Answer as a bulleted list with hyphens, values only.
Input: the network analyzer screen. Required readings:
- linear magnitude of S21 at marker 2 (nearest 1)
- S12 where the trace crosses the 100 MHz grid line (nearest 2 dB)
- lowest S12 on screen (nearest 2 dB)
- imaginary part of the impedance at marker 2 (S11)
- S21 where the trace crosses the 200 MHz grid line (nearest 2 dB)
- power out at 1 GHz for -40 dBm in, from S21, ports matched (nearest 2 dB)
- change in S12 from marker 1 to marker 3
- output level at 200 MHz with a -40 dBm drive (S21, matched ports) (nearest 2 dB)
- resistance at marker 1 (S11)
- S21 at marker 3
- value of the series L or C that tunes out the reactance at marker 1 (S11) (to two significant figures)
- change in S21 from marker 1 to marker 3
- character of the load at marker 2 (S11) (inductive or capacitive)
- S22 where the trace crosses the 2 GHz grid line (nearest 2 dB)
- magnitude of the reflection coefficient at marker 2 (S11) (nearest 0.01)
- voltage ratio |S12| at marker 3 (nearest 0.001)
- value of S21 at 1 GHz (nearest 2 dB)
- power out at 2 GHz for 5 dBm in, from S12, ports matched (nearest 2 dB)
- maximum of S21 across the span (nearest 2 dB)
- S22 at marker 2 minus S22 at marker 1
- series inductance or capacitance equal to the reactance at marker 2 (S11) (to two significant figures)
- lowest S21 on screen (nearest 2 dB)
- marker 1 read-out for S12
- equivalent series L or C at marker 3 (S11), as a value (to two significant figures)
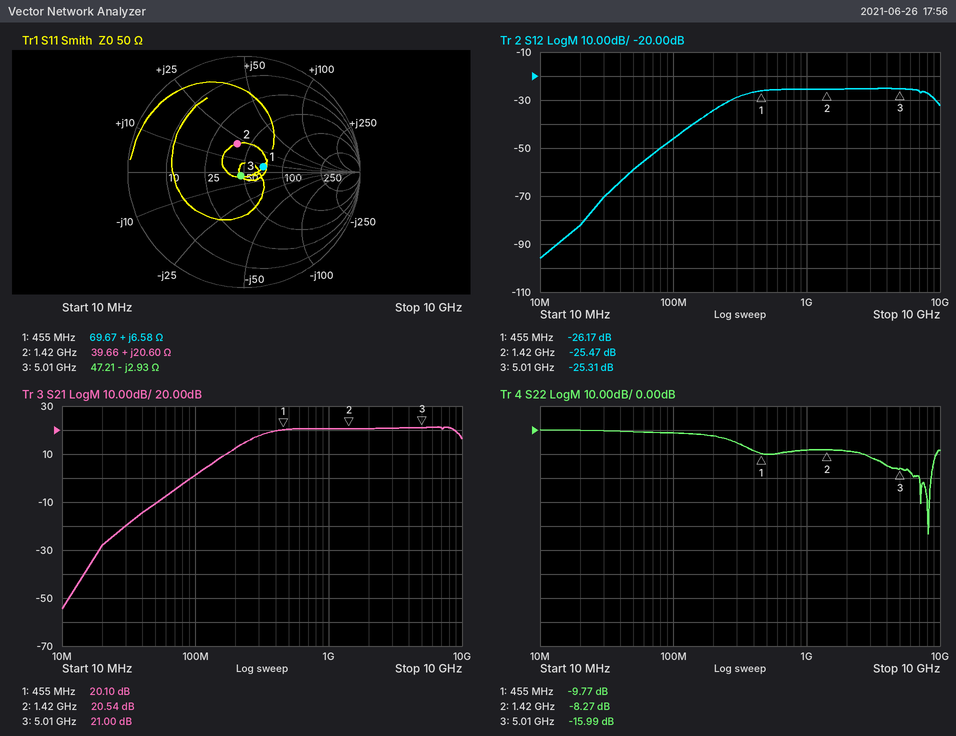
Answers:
- 11
- -46 dB
- -96 dB
- +20.60 Ω
- 12 dB
- -20 dBm
- 0.86 dB
- -28 dBm
- 69.67 Ω
- 21.00 dB
- 53 pF
- 0.90 dB
- inductive
- -8 dB
- 0.25
- 0.054
- 20 dB
- -20 dBm
- 22 dB
- 1.50 dB
- 2.3 nH
- -54 dB
- -26.17 dB
- 11 pF
